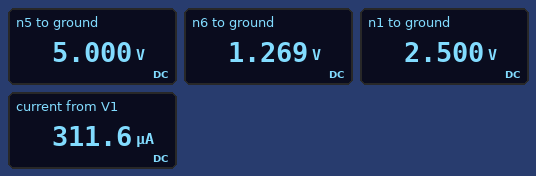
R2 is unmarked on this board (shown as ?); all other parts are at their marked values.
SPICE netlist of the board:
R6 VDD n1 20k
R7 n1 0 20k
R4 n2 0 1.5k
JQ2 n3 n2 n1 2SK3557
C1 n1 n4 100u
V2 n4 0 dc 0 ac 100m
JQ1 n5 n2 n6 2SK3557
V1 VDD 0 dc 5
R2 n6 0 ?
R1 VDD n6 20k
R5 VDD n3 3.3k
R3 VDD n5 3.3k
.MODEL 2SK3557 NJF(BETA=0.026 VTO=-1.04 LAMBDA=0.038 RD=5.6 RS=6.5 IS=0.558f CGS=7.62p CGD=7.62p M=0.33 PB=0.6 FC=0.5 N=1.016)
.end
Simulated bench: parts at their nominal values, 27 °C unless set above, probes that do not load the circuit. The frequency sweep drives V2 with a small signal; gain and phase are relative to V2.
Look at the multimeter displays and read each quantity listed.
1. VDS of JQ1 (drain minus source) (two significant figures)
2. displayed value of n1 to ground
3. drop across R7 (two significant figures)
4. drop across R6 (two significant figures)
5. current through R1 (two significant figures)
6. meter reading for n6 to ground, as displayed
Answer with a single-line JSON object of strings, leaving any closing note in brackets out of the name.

{"VDS of JQ1 (drain minus source)": "3.7 V", "displayed value of n1 to ground": "2.500 V", "drop across R7": "2.5 V", "drop across R6": "2.5 V", "current through R1": "190 µA", "meter reading for n6 to ground, as displayed": "1.269 V"}
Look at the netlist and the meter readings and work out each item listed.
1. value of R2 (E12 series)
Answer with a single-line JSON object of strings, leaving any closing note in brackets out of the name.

{"value of R2": "6.8 kΩ"}
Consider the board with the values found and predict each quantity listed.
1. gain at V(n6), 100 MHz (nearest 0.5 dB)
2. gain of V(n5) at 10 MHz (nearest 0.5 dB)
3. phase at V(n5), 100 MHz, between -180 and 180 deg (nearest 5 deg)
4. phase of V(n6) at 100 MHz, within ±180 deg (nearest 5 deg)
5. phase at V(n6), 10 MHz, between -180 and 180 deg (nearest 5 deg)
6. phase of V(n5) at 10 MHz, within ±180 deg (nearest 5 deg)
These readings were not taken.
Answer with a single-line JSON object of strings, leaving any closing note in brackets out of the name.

{"gain at V(n6), 100 MHz": "-2.0 dB", "gain of V(n5) at 10 MHz": "-21.0 dB", "phase at V(n5), 100 MHz, between -180 and 180 deg": "45 deg", "phase of V(n6) at 100 MHz, within ±180 deg": "35 deg", "phase at V(n6), 10 MHz, between -180 and 180 deg": "95 deg", "phase of V(n5) at 10 MHz, within ±180 deg": "120 deg"}
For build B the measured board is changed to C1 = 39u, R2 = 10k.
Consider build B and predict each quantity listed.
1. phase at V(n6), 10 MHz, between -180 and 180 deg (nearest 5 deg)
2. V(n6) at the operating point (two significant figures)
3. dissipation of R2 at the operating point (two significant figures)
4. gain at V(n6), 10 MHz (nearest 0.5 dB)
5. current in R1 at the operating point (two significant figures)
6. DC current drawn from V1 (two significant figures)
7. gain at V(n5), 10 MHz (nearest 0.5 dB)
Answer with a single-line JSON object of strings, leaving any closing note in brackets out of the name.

{"phase at V(n6), 10 MHz, between -180 and 180 deg": "90 deg", "V(n6) at the operating point": "1.7 V", "dissipation of R2 at the operating point": "280 µW", "gain at V(n6), 10 MHz": "-15.5 dB", "current in R1 at the operating point": "170 µA", "DC current drawn from V1": "290 µA", "gain at V(n5), 10 MHz": "-20.5 dB"}
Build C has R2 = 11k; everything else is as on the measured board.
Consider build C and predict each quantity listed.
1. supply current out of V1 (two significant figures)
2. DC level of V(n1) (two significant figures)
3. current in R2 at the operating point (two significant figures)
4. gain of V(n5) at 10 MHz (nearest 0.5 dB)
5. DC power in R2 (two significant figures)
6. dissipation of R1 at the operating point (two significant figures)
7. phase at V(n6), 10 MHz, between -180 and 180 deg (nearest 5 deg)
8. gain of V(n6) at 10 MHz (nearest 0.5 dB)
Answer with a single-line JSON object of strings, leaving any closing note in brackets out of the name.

{"supply current out of V1": "290 µA", "DC level of V(n1)": "2.5 V", "current in R2 at the operating point": "160 µA", "gain of V(n5) at 10 MHz": "-20.5 dB", "DC power in R2": "290 µW", "dissipation of R1 at the operating point": "520 µW", "phase at V(n6), 10 MHz, between -180 and 180 deg": "90 deg", "gain of V(n6) at 10 MHz": "-15.0 dB"}
